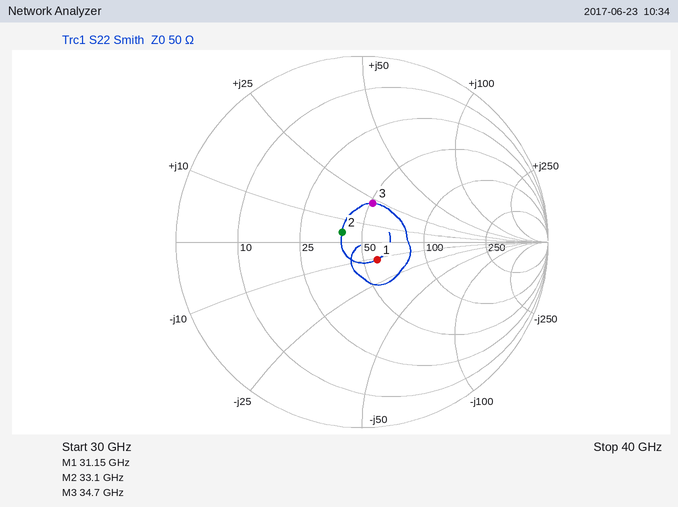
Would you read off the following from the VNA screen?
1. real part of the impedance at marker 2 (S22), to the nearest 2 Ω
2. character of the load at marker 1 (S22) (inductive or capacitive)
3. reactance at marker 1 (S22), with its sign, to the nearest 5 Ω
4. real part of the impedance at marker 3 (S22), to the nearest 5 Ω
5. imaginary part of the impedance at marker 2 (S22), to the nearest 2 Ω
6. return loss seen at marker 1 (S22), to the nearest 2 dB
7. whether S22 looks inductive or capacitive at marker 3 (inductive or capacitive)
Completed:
40 Ω
capacitive
-10 Ω
50 Ω
+4 Ω
18 dB
inductive
